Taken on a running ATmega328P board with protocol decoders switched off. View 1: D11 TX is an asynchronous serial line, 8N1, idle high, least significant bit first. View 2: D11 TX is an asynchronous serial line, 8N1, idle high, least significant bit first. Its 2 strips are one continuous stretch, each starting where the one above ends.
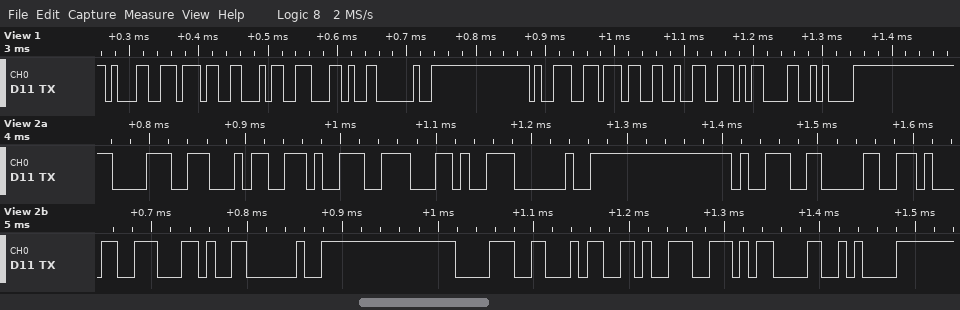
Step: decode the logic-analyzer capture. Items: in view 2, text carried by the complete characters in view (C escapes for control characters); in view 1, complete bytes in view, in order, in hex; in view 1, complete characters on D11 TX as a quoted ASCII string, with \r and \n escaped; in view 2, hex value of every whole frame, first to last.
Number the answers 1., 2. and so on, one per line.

1. "849, 901, 849\r\n"
2. 0x31 0x37 0x34 0x2C 0x20 0x39 0x37 0x32 0x0D 0x0A
3. "174, 972\r\n"
4. 38 34 39 2C 20 39 30 31 2C 20 38 34 39 0D 0A
